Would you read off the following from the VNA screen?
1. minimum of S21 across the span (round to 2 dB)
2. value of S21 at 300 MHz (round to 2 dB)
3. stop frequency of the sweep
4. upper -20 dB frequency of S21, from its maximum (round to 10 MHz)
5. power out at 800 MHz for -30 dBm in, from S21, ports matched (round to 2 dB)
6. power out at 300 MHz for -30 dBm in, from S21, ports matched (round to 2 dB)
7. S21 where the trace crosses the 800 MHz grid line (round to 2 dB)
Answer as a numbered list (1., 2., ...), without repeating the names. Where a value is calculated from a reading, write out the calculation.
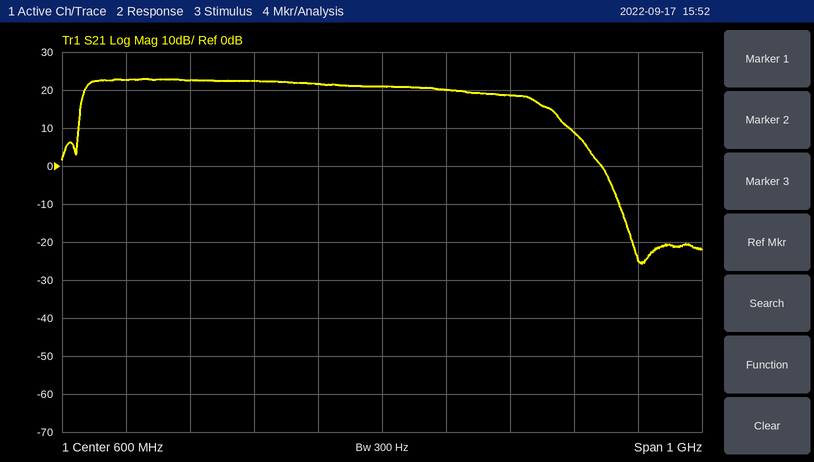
1. -26 dB
2. 22 dB
3. 1.1 GHz
4. 930 MHz
5. -30 dBm + (18 dB) = -12 dBm
6. -30 dBm + (22 dB) = -8 dBm
7. 18 dB
